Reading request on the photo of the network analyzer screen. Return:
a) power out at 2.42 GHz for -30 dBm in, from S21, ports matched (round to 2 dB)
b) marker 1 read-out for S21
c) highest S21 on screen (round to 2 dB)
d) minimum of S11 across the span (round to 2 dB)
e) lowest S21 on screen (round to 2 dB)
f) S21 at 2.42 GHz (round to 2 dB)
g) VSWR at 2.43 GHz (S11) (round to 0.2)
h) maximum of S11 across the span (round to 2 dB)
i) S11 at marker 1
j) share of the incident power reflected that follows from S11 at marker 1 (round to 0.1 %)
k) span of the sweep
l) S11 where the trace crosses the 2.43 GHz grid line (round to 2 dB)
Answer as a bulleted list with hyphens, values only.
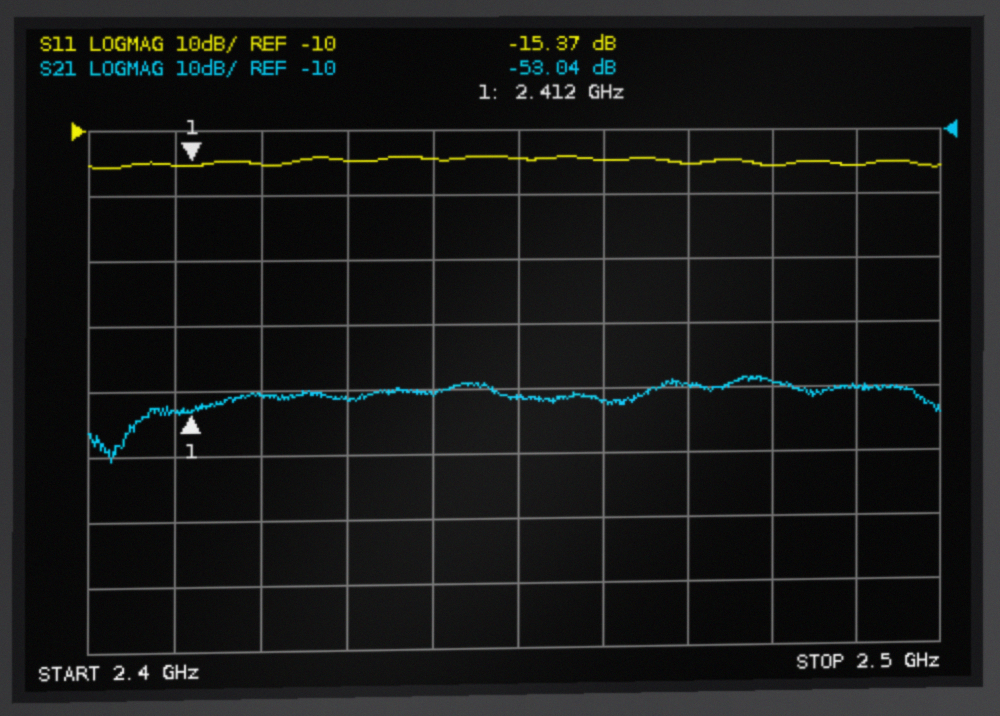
- -80 dBm
- -53.04 dB
- -48 dB
- -16 dB
- -60 dB
- -50 dB
- 1.4
- -14 dB
- -15.37 dB
- 2.9 %
- 100 MHz
- -14 dB
